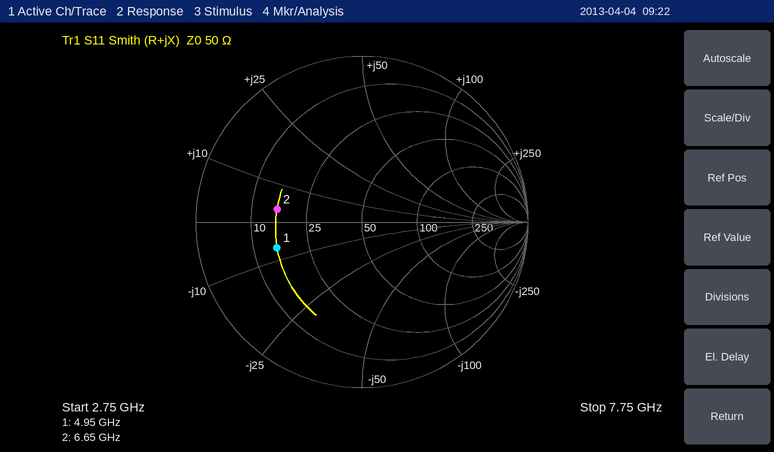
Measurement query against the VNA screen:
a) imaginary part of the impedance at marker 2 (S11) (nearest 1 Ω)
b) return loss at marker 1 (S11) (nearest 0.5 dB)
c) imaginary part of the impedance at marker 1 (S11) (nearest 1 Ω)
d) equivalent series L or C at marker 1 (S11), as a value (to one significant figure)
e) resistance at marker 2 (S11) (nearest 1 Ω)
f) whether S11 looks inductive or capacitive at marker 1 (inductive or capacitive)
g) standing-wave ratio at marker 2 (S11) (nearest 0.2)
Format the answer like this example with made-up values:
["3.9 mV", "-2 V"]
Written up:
["+3 Ω", "5.5 dB", "-7 Ω", "5 pF", "16 Ω", "capacitive", "3.2"]
